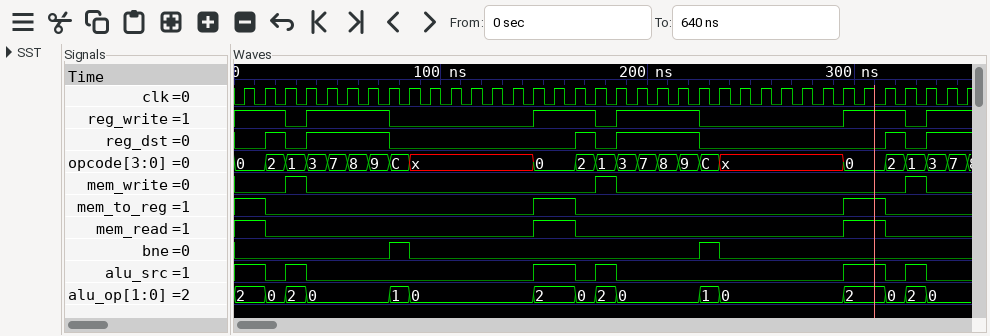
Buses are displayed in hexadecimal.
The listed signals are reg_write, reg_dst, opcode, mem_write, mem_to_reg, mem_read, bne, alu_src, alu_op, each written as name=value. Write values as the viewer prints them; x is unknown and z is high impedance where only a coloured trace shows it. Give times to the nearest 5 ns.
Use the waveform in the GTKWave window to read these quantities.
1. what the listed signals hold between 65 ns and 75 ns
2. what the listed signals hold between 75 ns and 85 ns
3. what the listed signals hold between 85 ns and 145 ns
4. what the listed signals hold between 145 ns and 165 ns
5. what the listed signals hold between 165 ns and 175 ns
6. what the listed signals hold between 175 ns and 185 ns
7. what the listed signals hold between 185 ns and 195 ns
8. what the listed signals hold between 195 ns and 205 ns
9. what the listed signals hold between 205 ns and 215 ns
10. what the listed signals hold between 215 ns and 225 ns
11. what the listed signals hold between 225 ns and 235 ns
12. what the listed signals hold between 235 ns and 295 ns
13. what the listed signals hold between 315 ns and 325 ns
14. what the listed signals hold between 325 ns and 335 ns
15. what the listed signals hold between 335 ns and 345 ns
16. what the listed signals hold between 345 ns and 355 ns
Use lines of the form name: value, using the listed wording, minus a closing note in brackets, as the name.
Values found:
what the listed signals hold between 65 ns and 75 ns: reg_write=1, reg_dst=1, opcode=9, mem_write=0, mem_to_reg=0, mem_read=0, bne=0, alu_src=0, alu_op=0
what the listed signals hold between 75 ns and 85 ns: reg_write=0, reg_dst=0, opcode=C, mem_write=0, mem_to_reg=0, mem_read=0, bne=1, alu_src=0, alu_op=1
what the listed signals hold between 85 ns and 145 ns: reg_write=0, reg_dst=0, opcode=x, mem_write=0, mem_to_reg=0, mem_read=0, bne=0, alu_src=0, alu_op=0
what the listed signals hold between 145 ns and 165 ns: reg_write=1, reg_dst=0, opcode=0, mem_write=0, mem_to_reg=1, mem_read=1, bne=0, alu_src=1, alu_op=2
what the listed signals hold between 165 ns and 175 ns: reg_write=1, reg_dst=1, opcode=2, mem_write=0, mem_to_reg=0, mem_read=0, bne=0, alu_src=0, alu_op=0
what the listed signals hold between 175 ns and 185 ns: reg_write=0, reg_dst=0, opcode=1, mem_write=1, mem_to_reg=0, mem_read=0, bne=0, alu_src=1, alu_op=2
what the listed signals hold between 185 ns and 195 ns: reg_write=1, reg_dst=1, opcode=3, mem_write=0, mem_to_reg=0, mem_read=0, bne=0, alu_src=0, alu_op=0
what the listed signals hold between 195 ns and 205 ns: reg_write=1, reg_dst=1, opcode=7, mem_write=0, mem_to_reg=0, mem_read=0, bne=0, alu_src=0, alu_op=0
what the listed signals hold between 205 ns and 215 ns: reg_write=1, reg_dst=1, opcode=8, mem_write=0, mem_to_reg=0, mem_read=0, bne=0, alu_src=0, alu_op=0
what the listed signals hold between 215 ns and 225 ns: reg_write=1, reg_dst=1, opcode=9, mem_write=0, mem_to_reg=0, mem_read=0, bne=0, alu_src=0, alu_op=0
what the listed signals hold between 225 ns and 235 ns: reg_write=0, reg_dst=0, opcode=C, mem_write=0, mem_to_reg=0, mem_read=0, bne=1, alu_src=0, alu_op=1
what the listed signals hold between 235 ns and 295 ns: reg_write=0, reg_dst=0, opcode=x, mem_write=0, mem_to_reg=0, mem_read=0, bne=0, alu_src=0, alu_op=0
what the listed signals hold between 315 ns and 325 ns: reg_write=1, reg_dst=1, opcode=2, mem_write=0, mem_to_reg=0, mem_read=0, bne=0, alu_src=0, alu_op=0
what the listed signals hold between 325 ns and 335 ns: reg_write=0, reg_dst=0, opcode=1, mem_write=1, mem_to_reg=0, mem_read=0, bne=0, alu_src=1, alu_op=2
what the listed signals hold between 335 ns and 345 ns: reg_write=1, reg_dst=1, opcode=3, mem_write=0, mem_to_reg=0, mem_read=0, bne=0, alu_src=0, alu_op=0
what the listed signals hold between 345 ns and 355 ns: reg_write=1, reg_dst=1, opcode=7, mem_write=0, mem_to_reg=0, mem_read=0, bne=0, alu_src=0, alu_op=0
